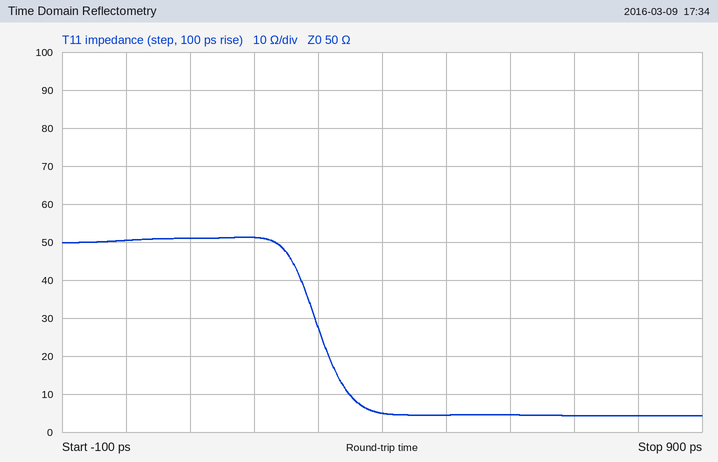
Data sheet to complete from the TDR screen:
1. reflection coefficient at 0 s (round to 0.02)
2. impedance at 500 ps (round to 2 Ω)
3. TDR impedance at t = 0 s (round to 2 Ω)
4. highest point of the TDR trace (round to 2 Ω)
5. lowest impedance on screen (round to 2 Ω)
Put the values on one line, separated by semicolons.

0.00; 4 Ω; 50 Ω; 52 Ω; 4 Ω
